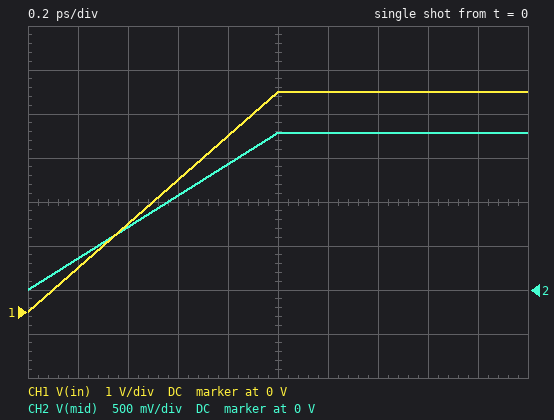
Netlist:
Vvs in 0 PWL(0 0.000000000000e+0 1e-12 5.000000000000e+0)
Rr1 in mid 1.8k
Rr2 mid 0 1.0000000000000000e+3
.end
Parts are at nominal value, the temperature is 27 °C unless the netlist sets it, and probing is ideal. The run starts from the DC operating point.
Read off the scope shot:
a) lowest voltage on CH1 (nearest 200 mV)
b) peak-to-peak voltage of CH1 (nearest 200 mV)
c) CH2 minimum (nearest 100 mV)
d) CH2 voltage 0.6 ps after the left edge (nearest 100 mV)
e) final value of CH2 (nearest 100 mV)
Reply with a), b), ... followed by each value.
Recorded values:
a) 0 V
b) 5.0 V
c) 0 V
d) 1.1 V
e) 1.8 V
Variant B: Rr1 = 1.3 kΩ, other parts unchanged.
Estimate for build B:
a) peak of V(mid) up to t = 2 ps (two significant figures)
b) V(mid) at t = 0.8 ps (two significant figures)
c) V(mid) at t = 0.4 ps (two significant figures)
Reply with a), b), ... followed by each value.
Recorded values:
a) 2.2 V
b) 1.7 V
c) 870 mV
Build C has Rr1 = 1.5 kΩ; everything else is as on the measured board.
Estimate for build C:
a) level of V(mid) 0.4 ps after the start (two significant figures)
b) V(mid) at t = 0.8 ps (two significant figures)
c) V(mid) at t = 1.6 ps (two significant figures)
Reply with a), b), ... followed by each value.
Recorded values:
a) 800 mV
b) 1.6 V
c) 2.0 V
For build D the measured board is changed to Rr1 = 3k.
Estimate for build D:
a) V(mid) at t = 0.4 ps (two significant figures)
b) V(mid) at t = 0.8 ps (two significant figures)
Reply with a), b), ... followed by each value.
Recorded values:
a) 500 mV
b) 1.0 V
